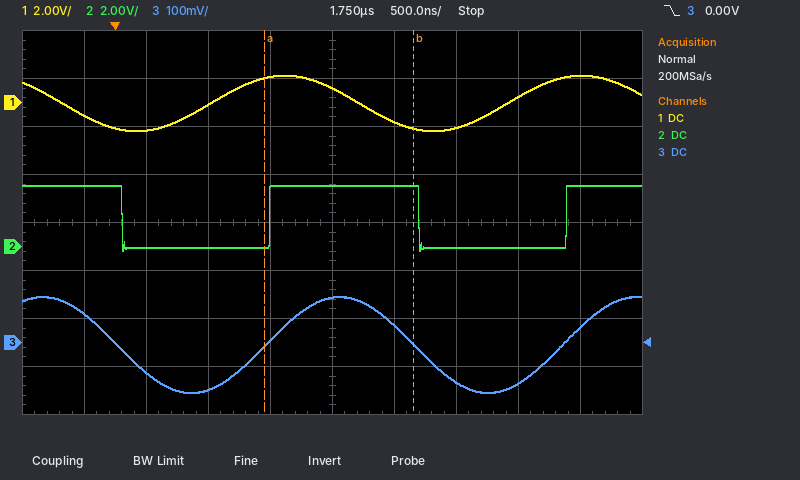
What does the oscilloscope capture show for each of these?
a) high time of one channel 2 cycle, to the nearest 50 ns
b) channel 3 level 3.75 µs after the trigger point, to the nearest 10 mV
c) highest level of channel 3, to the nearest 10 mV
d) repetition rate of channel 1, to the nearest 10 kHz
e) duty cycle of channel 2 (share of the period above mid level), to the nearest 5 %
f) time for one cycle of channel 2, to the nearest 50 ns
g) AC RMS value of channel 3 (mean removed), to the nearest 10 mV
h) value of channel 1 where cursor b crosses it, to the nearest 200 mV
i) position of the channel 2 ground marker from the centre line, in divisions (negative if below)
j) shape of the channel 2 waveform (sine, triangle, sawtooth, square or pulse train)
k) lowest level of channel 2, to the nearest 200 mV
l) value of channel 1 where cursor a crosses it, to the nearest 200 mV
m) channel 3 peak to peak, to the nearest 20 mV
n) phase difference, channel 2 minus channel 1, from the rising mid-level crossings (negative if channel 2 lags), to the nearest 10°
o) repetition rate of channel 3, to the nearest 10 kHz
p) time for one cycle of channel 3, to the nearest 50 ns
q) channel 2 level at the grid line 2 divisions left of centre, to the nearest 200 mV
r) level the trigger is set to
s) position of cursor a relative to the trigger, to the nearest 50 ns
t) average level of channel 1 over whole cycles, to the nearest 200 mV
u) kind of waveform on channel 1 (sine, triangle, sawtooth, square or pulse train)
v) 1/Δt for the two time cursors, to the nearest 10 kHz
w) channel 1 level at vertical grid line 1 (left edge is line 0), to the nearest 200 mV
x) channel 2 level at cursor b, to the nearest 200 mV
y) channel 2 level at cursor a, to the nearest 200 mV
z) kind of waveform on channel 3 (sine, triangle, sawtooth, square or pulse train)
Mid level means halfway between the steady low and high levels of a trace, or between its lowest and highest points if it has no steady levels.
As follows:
1.20 µs
30 mV
100 mV
420 kHz
50 %
2.40 µs
70 mV
-1.0 V
-0.5 div
square
-200 mV
1.0 V
200 mV
-70°
420 kHz
2.40 µs
0.0 V
0.00 V
+1.20 µs
0.0 V
sine
830 kHz
-600 mV
2.6 V
0.0 V
sine
